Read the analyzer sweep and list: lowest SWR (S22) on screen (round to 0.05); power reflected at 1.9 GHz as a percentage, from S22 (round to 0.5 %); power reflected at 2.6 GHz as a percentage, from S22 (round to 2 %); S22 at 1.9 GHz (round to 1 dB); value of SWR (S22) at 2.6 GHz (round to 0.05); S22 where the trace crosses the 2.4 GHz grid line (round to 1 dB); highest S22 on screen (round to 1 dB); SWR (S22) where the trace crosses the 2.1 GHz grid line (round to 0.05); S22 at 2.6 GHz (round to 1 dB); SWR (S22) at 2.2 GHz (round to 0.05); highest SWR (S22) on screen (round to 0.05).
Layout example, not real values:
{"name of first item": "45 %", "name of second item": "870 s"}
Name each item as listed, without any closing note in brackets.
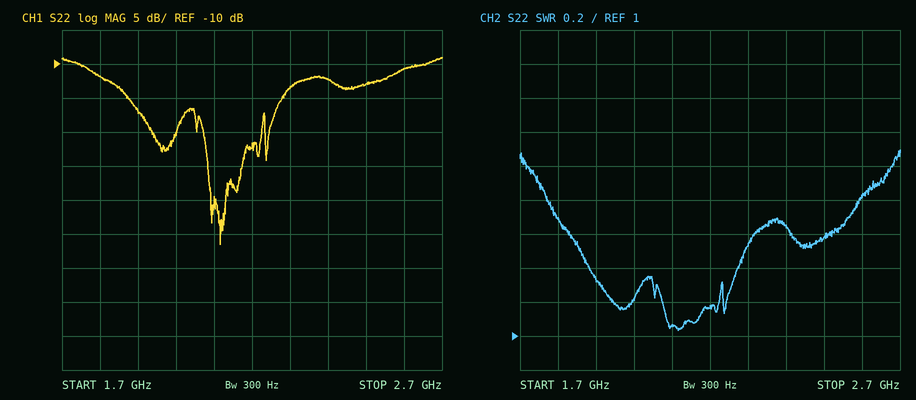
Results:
{"lowest SWR (S22) on screen": "1.05", "power reflected at 1.9 GHz as a percentage, from S22": "2.0 %", "power reflected at 2.6 GHz as a percentage, from S22": "8 %", "S22 at 1.9 GHz": "-17 dB", "value of SWR (S22) at 2.6 GHz": "1.80", "S22 where the trace crosses the 2.4 GHz grid line": "-12 dB", "highest S22 on screen": "-9 dB", "SWR (S22) where the trace crosses the 2.1 GHz grid line": "1.05", "S22 at 2.6 GHz": "-11 dB", "SWR (S22) at 2.2 GHz": "1.15", "highest SWR (S22) on screen": "2.10"}
